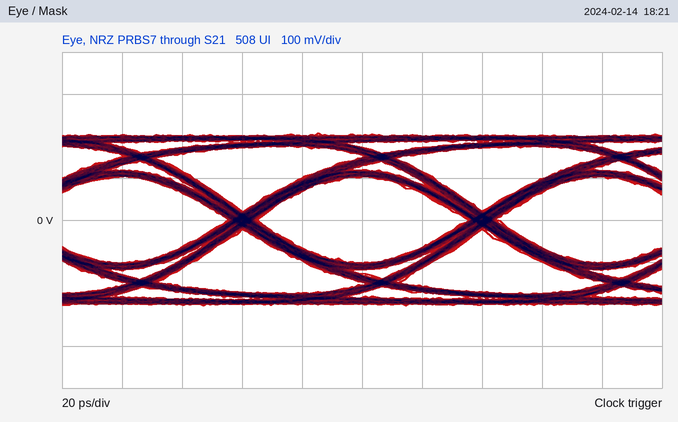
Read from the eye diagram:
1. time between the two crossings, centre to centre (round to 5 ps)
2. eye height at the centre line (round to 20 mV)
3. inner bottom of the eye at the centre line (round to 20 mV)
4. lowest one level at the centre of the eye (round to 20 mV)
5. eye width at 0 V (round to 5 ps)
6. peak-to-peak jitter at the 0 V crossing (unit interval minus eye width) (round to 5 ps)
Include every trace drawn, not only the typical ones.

80 ps
200 mV
-100 mV
100 mV
70 ps
10 ps
